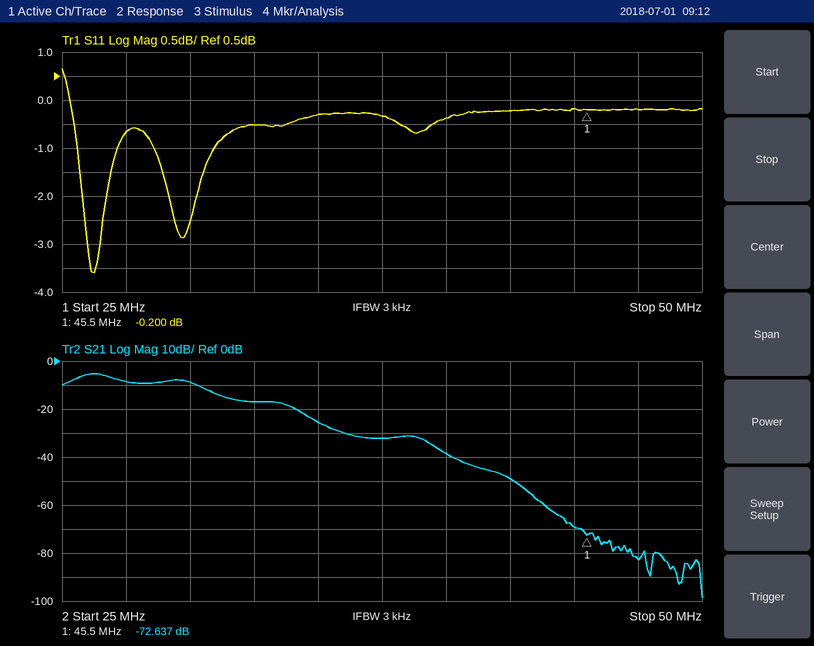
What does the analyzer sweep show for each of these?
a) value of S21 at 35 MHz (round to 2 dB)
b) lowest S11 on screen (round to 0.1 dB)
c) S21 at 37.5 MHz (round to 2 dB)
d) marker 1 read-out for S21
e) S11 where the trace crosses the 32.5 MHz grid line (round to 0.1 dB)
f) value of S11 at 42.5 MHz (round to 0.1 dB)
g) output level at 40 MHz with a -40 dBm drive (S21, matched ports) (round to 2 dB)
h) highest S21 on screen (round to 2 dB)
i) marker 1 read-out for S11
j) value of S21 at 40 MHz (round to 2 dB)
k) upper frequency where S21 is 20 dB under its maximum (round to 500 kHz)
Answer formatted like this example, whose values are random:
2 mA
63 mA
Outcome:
-26 dB
-3.6 dB
-32 dB
-72.637 dB
-0.5 dB
-0.2 dB
-78 dBm
-6 dB
-0.200 dB
-38 dB
35.0 MHz
